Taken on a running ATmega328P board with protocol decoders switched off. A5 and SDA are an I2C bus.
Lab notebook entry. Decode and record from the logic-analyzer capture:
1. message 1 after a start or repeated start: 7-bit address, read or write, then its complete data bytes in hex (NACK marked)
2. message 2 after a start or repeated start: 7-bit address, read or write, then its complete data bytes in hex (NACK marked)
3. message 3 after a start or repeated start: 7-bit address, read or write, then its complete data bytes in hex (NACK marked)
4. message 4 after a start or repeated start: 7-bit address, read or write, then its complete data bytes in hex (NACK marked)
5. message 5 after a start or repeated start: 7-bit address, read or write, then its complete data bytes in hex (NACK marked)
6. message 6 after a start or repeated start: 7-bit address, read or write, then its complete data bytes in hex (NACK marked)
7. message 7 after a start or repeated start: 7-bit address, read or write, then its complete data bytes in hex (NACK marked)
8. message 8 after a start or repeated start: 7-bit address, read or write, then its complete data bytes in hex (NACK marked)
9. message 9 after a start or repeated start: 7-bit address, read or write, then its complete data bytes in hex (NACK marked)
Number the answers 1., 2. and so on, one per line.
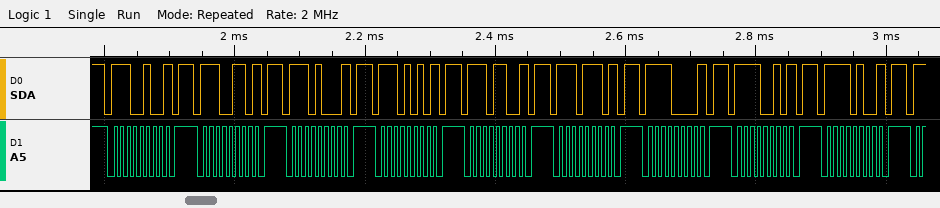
1. 0x72 write NACK
2. 0x73 write NACK
3. 0x74 write NACK
4. 0x75 write NACK
5. 0x76 write NACK
6. 0x77 write NACK
7. 0x78 write NACK
8. 0x79 write NACK
9. 0x7A write NACK
